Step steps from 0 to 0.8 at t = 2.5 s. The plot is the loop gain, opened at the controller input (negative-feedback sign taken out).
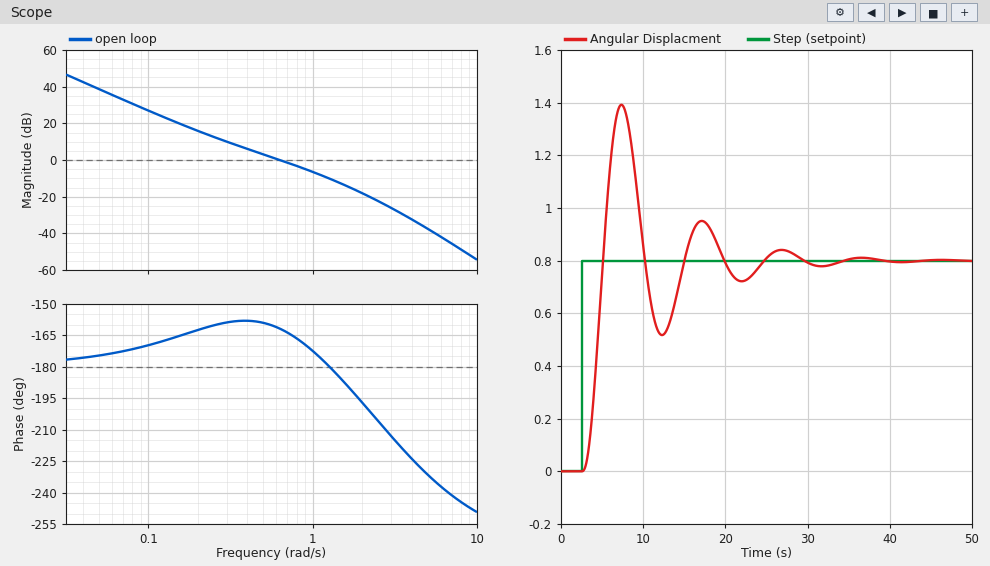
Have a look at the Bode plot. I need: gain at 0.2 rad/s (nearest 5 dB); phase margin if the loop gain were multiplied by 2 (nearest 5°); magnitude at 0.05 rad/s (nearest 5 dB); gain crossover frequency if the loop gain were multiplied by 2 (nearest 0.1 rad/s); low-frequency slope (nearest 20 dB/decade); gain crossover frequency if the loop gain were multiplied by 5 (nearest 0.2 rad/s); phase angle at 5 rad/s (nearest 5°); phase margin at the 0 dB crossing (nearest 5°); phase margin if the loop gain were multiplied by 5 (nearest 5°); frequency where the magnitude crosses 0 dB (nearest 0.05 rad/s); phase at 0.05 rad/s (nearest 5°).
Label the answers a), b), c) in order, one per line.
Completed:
a) 15 dB
b) 10°
c) 40 dB
d) 1.0 rad/s
e) -40 dB/decade
f) 1.6 rad/s
g) -230°
h) 20°
i) -10°
j) 0.65 rad/s
k) -175°
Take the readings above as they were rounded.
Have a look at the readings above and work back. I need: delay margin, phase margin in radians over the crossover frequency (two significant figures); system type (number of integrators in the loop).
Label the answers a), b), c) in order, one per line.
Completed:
a) 0.54 s
b) 2
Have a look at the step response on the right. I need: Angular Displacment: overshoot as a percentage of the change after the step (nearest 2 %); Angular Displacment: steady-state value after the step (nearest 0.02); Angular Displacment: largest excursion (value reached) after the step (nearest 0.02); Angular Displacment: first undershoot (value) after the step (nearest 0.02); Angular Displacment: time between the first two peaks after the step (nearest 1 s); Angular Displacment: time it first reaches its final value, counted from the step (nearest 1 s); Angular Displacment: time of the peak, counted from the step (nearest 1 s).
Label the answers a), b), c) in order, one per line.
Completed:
a) 74 %
b) 0.80
c) 1.40
d) 0.52
e) 10 s
f) 3 s
g) 5 s
